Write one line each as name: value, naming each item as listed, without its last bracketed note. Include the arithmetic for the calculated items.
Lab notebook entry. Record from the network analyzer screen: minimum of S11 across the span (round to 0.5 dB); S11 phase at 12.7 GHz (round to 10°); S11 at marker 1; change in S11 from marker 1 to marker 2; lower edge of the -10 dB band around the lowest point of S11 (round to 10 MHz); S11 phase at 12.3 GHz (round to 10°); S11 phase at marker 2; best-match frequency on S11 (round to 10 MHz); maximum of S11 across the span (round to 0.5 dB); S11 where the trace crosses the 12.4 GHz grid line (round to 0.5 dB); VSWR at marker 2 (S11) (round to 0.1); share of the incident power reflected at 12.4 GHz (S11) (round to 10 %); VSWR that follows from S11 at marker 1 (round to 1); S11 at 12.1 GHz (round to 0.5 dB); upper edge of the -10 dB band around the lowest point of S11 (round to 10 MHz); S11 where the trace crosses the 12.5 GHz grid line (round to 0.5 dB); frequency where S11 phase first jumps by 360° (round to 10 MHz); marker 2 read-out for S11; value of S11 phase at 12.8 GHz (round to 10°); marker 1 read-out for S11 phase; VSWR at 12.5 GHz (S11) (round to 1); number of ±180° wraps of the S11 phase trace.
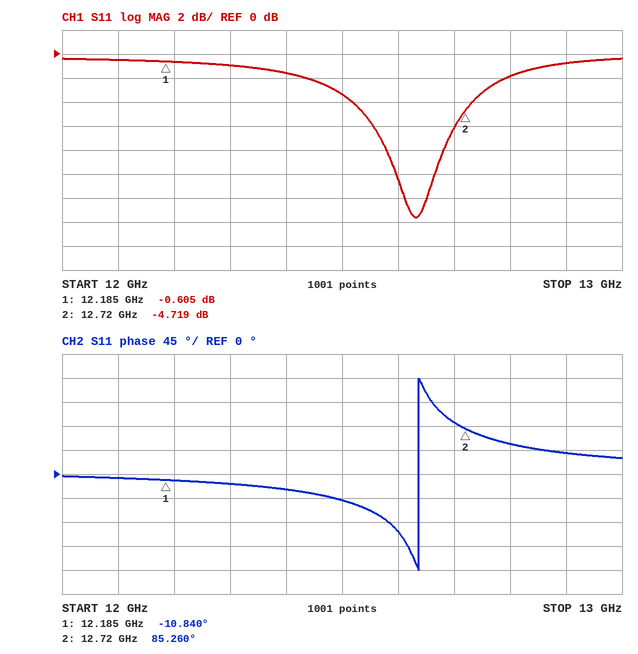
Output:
minimum of S11 across the span: -13.5 dB
S11 phase at 12.7 GHz: 100°
S11 at marker 1: -0.605 dB
change in S11 from marker 1 to marker 2: -4.719 − (-0.605) = -4.114 dB
lower edge of the -10 dB band around the lowest point of S11: 12.60 GHz
S11 phase at 12.3 GHz: -20°
S11 phase at marker 2: 85.260°
best-match frequency on S11: 12.63 GHz
maximum of S11 across the span: -0.5 dB
S11 where the trace crosses the 12.4 GHz grid line: -1.5 dB
VSWR at marker 2 (S11): (1 + 0.5808)/(1 − 0.5808) ≈ 3.8
share of the incident power reflected at 12.4 GHz (S11): 10^(-1.5/10) ≈ 70.8 %, so 70 % to the nearest 10 %
VSWR that follows from S11 at marker 1: (1 + 0.9327)/(1 − 0.9327) ≈ 29
S11 at 12.1 GHz: -0.5 dB
upper edge of the -10 dB band around the lowest point of S11: 12.67 GHz
S11 where the trace crosses the 12.5 GHz grid line: -3.5 dB
frequency where S11 phase first jumps by 360°: 12.64 GHz
marker 2 read-out for S11: -4.719 dB
value of S11 phase at 12.8 GHz: 60°
marker 1 read-out for S11 phase: -10.840°
VSWR at 12.5 GHz (S11): |Γ| = 10^(-3.5/20) = 0.6683; VSWR = (1 + 0.6683)/(1 − 0.6683) ≈ 5
number of ±180° wraps of the S11 phase trace: 1
